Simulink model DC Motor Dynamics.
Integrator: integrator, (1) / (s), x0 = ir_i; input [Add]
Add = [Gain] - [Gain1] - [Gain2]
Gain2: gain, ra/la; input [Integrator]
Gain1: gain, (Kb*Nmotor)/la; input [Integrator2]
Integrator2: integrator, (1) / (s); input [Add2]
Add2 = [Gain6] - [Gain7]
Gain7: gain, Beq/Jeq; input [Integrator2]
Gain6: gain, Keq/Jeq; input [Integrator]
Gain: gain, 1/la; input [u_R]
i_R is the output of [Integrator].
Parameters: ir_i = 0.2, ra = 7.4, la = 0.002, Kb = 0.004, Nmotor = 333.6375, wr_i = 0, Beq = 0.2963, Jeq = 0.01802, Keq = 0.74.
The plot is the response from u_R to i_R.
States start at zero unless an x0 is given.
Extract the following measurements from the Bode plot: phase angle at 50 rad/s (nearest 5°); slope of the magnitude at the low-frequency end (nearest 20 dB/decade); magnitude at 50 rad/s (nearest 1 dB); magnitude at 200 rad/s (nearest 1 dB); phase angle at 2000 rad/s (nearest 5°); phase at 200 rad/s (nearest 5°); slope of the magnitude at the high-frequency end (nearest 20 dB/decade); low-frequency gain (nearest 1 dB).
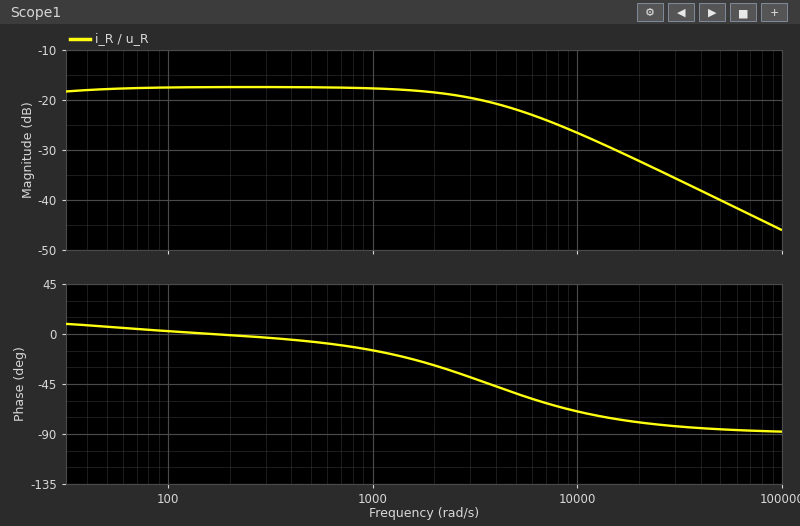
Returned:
5°
0 dB/decade
-18 dB
-17 dB
-30°
0°
-20 dB/decade
-18 dB
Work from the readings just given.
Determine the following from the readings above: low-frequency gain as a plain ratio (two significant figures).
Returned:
0.13
